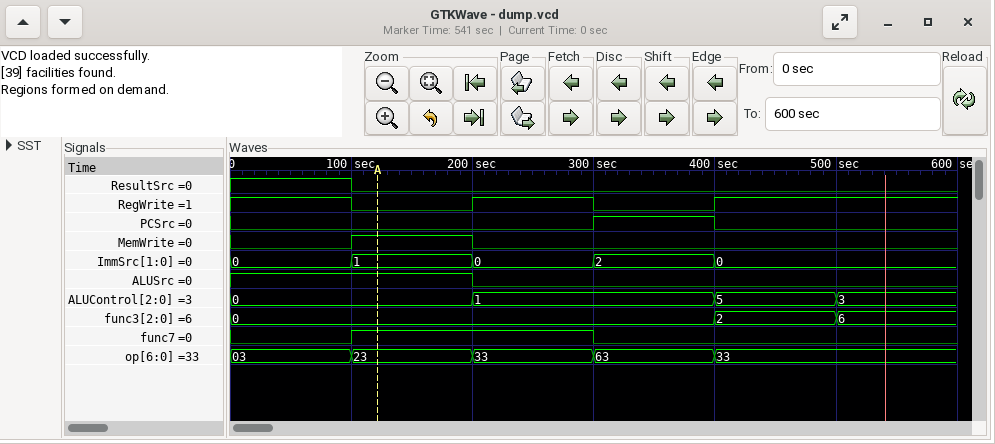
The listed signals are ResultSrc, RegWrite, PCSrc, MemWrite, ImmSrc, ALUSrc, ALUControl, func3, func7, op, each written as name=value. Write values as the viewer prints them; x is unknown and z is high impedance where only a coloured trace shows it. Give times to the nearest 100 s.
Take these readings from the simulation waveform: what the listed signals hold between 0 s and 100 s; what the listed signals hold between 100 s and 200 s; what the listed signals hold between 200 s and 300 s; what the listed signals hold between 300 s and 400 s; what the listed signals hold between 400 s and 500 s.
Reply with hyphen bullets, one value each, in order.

- ResultSrc=1, RegWrite=1, PCSrc=0, MemWrite=0, ImmSrc=0, ALUSrc=1, ALUControl=0, func3=0, func7=0, op=03
- ResultSrc=0, RegWrite=0, PCSrc=0, MemWrite=1, ImmSrc=1, ALUSrc=1, ALUControl=0, func3=0, func7=1, op=23
- ResultSrc=0, RegWrite=1, PCSrc=0, MemWrite=0, ImmSrc=0, ALUSrc=0, ALUControl=1, func3=0, func7=1, op=33
- ResultSrc=0, RegWrite=0, PCSrc=1, MemWrite=0, ImmSrc=2, ALUSrc=0, ALUControl=1, func3=0, func7=0, op=63
- ResultSrc=0, RegWrite=1, PCSrc=0, MemWrite=0, ImmSrc=0, ALUSrc=0, ALUControl=5, func3=2, func7=0, op=33
